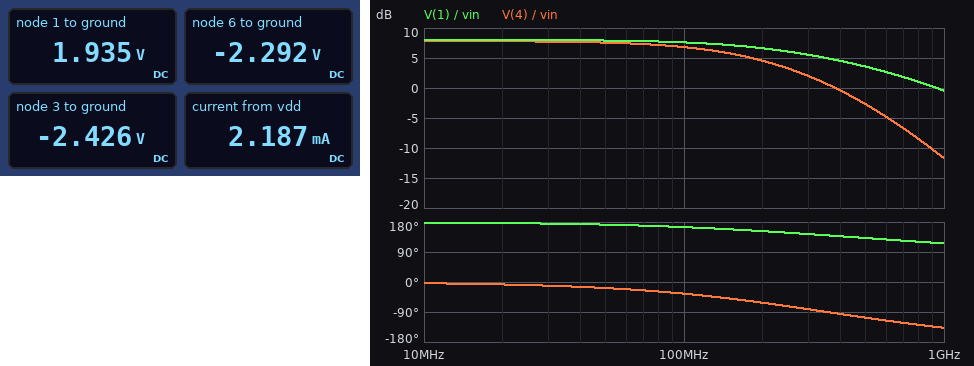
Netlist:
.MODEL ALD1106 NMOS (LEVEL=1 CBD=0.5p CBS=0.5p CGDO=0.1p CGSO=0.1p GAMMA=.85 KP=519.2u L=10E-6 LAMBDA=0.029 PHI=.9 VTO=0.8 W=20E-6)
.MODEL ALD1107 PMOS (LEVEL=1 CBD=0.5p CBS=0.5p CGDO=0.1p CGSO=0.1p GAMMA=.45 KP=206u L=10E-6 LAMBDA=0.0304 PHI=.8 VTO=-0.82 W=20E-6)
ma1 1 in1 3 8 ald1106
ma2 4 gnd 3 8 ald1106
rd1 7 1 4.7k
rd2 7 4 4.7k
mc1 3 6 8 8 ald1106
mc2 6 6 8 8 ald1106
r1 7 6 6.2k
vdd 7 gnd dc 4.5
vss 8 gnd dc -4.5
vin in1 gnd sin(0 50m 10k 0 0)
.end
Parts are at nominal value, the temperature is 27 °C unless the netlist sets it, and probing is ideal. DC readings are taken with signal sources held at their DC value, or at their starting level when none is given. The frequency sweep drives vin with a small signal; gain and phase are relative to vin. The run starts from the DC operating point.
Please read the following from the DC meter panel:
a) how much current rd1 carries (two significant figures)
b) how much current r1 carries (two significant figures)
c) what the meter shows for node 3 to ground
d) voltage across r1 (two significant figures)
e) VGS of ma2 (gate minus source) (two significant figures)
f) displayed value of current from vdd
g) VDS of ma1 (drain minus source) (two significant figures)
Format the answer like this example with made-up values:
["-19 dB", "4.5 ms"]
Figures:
["550 µA", "1.1 mA", "-2.426 V", "6.8 V", "2.4 V", "2.187 mA", "4.4 V"]
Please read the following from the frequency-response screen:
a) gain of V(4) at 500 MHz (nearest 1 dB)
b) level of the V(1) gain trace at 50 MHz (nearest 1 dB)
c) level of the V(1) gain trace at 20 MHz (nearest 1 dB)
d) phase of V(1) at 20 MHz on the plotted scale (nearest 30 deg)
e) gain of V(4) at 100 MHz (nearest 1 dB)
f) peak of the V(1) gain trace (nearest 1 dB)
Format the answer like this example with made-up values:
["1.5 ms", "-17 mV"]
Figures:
["-3 dB", "8 dB", "8 dB", "180 deg", "7 dB", "8 dB"]
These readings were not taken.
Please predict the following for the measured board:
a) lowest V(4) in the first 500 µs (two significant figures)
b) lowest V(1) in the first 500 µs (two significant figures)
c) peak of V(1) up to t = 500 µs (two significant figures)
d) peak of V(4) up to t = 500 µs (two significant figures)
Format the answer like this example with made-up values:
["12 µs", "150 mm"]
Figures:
["1.8 V", "1.8 V", "2.1 V", "2.1 V"]
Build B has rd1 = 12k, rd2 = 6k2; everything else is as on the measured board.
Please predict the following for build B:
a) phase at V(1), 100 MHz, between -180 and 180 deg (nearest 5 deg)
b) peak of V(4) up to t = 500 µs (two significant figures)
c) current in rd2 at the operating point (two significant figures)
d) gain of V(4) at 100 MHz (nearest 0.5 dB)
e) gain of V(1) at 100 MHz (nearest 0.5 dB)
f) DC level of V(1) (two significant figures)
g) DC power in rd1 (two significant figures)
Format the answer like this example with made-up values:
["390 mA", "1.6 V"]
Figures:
["150 deg", "970 mV", "580 µA", "2.5 dB", "4.5 dB", "-1.7 V", "3.2 mW"]
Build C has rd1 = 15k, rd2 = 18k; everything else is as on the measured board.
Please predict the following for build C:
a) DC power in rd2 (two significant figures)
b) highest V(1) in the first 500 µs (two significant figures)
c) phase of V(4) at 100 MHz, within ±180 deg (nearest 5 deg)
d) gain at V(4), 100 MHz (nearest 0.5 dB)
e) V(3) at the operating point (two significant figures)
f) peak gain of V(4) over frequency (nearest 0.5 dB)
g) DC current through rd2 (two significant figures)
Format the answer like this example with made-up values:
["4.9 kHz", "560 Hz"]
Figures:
["3.4 mW", "-3.3 V", "5 deg", "-35.0 dB", "-3.5 V", "-34.5 dB", "440 µA"]
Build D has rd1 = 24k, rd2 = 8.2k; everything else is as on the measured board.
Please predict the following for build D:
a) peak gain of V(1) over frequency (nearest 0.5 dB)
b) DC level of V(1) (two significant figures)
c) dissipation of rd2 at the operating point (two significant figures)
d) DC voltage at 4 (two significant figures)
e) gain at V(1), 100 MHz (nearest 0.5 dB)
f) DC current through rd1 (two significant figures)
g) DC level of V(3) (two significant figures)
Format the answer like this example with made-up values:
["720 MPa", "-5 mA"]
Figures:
["-16.0 dB", "-2.5 V", "5.1 mW", "-2.0 V", "-16.5 dB", "290 µA", "-2.7 V"]
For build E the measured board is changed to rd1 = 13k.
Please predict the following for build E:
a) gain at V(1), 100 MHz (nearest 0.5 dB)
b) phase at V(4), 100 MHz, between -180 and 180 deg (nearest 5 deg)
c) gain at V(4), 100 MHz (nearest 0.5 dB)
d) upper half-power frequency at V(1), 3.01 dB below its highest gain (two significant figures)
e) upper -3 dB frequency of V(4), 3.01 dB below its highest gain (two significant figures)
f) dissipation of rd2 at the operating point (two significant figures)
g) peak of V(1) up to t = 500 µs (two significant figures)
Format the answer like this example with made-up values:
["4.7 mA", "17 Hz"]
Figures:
["1.0 dB", "-5 deg", "-2.5 dB", "190 MHz", "350 MHz", "1.7 mW", "-1.7 V"]
